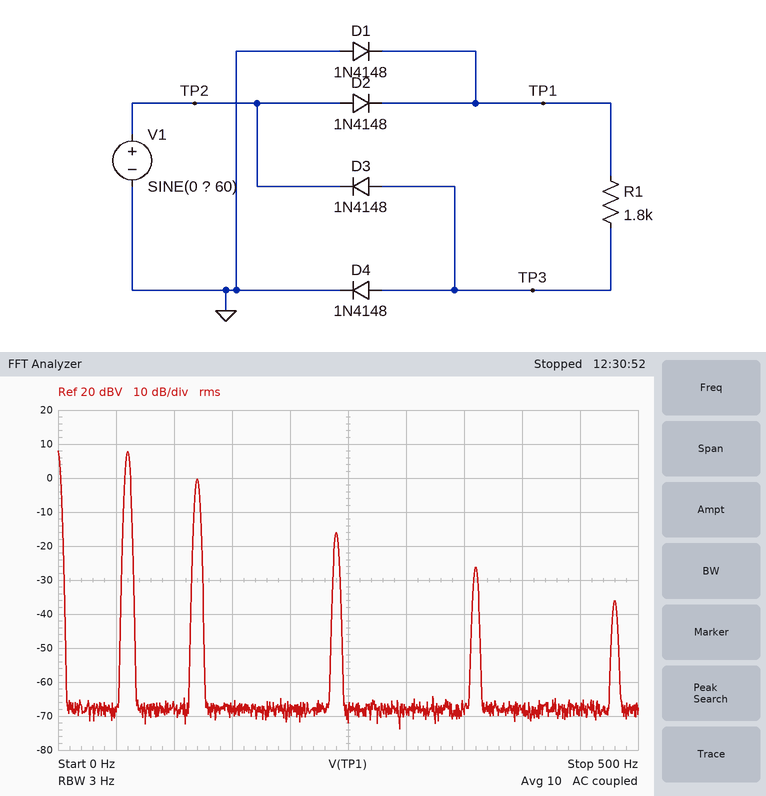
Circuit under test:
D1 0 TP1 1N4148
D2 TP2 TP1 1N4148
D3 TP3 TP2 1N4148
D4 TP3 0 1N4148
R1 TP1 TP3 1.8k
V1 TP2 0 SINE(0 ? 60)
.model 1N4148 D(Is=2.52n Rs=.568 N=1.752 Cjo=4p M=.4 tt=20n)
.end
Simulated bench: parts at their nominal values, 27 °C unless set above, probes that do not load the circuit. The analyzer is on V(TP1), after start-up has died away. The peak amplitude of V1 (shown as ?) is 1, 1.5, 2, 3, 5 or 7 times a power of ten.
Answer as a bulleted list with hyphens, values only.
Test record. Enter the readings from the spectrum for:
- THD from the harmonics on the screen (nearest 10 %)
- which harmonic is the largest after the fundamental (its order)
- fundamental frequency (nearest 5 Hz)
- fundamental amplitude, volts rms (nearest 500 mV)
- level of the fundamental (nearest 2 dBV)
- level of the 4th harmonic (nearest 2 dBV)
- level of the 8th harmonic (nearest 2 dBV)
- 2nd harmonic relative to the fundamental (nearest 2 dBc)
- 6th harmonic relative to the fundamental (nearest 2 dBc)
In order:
- 40 %
- 2
- 60 Hz
- 2.5 V
- 8 dBV
- -16 dBV
- -36 dBV
- -8 dBc
- -34 dBc
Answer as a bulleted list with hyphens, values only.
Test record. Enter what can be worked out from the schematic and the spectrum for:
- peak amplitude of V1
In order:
- 7 V
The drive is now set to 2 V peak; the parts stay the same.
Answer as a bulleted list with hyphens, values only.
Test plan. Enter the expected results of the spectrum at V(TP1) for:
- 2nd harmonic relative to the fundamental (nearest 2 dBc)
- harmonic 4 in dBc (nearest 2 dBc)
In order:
- -12 dBc
- -36 dBc
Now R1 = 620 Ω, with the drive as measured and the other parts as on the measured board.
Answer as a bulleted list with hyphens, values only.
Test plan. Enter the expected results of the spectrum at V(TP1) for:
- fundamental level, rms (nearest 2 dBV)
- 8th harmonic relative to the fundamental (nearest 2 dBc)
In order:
- 8 dBV
- -46 dBc
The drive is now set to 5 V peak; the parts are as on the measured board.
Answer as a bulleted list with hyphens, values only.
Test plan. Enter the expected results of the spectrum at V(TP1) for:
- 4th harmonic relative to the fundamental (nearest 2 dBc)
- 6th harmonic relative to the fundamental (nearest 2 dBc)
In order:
- -26 dBc
- -40 dBc
